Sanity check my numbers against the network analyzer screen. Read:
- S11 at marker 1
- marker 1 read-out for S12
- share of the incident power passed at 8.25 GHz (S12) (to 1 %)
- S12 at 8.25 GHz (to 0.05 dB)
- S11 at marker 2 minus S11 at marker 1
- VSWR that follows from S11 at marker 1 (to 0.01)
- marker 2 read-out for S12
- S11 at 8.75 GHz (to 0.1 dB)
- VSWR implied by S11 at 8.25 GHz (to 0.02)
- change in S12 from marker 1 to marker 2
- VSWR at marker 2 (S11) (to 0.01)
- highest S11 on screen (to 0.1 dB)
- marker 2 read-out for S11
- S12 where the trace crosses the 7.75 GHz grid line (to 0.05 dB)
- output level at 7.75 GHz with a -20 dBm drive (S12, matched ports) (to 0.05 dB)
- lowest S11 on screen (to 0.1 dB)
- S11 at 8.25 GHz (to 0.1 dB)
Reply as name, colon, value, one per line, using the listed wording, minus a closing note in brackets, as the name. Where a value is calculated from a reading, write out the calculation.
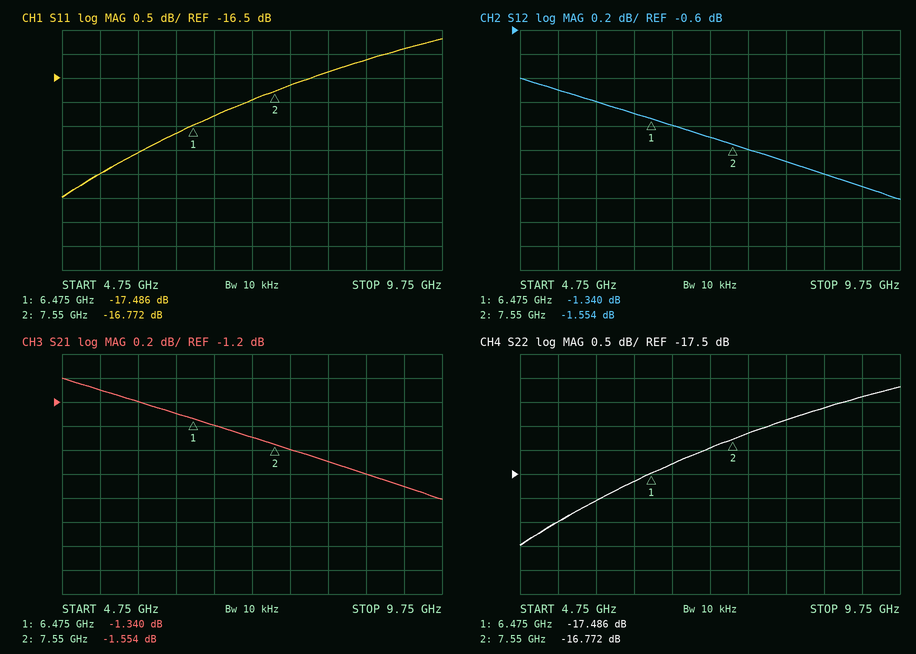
S11 at marker 1: -17.486 dB
marker 1 read-out for S12: -1.340 dB
share of the incident power passed at 8.25 GHz (S12): 10^(-1.7/10) ≈ 68 %
S12 at 8.25 GHz: -1.70 dB
S11 at marker 2 minus S11 at marker 1: -16.772 − (-17.486) = 0.714 dB
VSWR that follows from S11 at marker 1: (1 + 0.1336)/(1 − 0.1336) ≈ 1.31
marker 2 read-out for S12: -1.554 dB
S11 at 8.75 GHz: -16.1 dB
VSWR implied by S11 at 8.25 GHz: |Γ| = 10^(-16.4/20) = 0.1514; VSWR = (1 + 0.1514)/(1 − 0.1514) ≈ 1.36
change in S12 from marker 1 to marker 2: -1.554 − (-1.34) = -0.214 dB
VSWR at marker 2 (S11): (1 + 0.1450)/(1 − 0.1450) ≈ 1.34
highest S11 on screen: -15.7 dB
marker 2 read-out for S11: -16.772 dB
S12 where the trace crosses the 7.75 GHz grid line: -1.60 dB
output level at 7.75 GHz with a -20 dBm drive (S12, matched ports): -20 dBm + (-1.60 dB) = -21.60 dBm
lowest S11 on screen: -19.0 dB
S11 at 8.25 GHz: -16.4 dB
